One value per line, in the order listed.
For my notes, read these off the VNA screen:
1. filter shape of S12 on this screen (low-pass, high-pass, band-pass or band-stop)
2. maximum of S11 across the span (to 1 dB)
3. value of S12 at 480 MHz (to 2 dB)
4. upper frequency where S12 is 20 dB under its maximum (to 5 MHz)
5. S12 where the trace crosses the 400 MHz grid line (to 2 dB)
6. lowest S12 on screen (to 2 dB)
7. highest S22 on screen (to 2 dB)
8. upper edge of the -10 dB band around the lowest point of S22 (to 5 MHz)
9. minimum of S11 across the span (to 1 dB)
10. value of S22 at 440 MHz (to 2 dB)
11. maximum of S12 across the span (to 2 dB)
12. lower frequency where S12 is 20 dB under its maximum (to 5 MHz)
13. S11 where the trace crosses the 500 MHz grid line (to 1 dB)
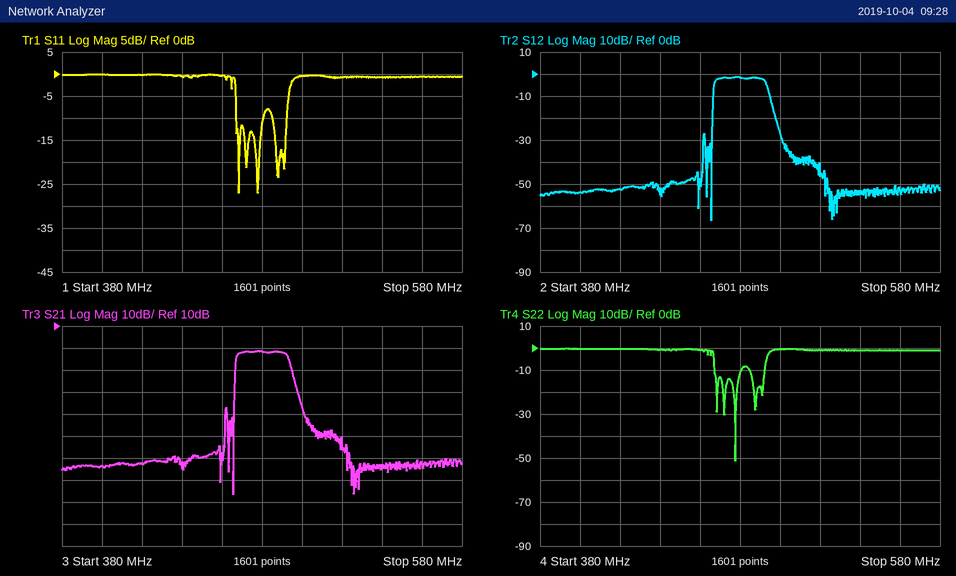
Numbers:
band-pass
0 dB
-2 dB
500 MHz
-54 dB
-66 dB
0 dB
480 MHz
-27 dB
0 dB
-2 dB
465 MHz
0 dB
